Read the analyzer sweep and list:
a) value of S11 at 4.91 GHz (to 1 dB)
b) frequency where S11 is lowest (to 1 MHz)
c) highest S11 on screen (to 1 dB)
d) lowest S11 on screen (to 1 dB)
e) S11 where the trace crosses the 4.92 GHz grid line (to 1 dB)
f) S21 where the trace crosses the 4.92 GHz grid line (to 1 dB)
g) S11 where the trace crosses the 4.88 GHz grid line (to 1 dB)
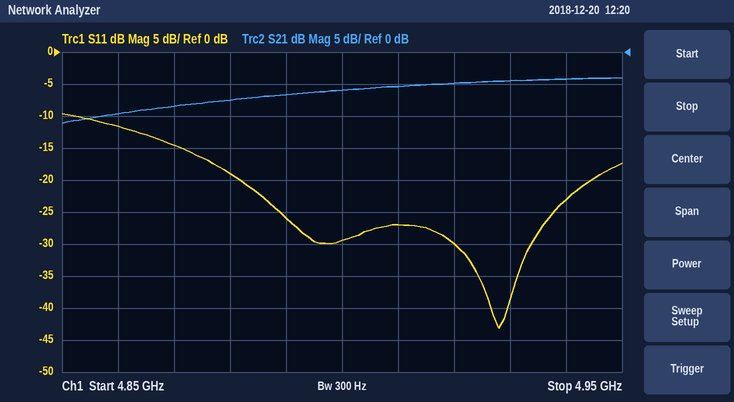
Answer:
-27 dB
4.928 GHz
-10 dB
-43 dB
-30 dB
-5 dB
-19 dB
